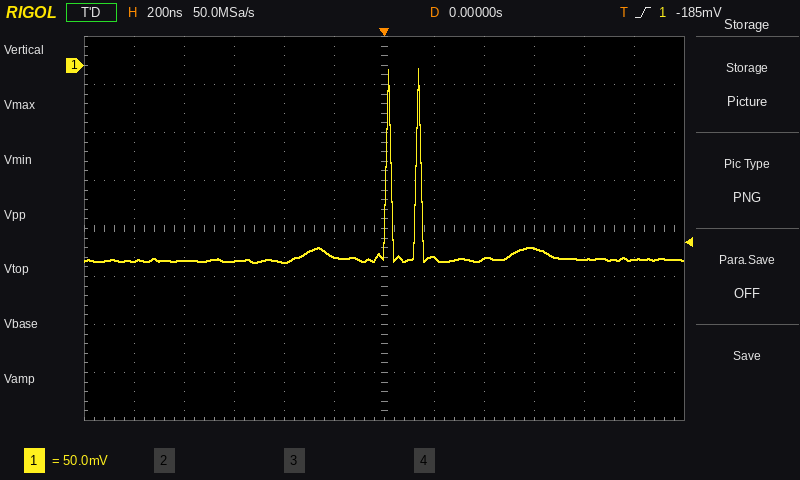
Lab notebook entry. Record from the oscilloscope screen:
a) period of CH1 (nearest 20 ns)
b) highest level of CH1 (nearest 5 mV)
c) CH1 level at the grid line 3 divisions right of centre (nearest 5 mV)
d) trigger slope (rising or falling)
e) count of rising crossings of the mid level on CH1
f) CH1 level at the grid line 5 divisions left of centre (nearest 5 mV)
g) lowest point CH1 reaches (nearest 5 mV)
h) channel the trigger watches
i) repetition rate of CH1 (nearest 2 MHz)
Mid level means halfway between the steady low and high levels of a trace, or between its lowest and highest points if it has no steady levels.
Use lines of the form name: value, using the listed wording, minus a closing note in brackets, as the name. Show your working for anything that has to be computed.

period of CH1: 120 ns
highest level of CH1: -5 mV
CH1 level at the grid line 3 divisions right of centre: -190 mV
trigger slope: rising
count of rising crossings of the mid level on CH1: 2
CH1 level at the grid line 5 divisions left of centre: -205 mV
lowest point CH1 reaches: -205 mV
channel the trigger watches: CH1
repetition rate of CH1: 1 / 120 ns ≈ 8 MHz
